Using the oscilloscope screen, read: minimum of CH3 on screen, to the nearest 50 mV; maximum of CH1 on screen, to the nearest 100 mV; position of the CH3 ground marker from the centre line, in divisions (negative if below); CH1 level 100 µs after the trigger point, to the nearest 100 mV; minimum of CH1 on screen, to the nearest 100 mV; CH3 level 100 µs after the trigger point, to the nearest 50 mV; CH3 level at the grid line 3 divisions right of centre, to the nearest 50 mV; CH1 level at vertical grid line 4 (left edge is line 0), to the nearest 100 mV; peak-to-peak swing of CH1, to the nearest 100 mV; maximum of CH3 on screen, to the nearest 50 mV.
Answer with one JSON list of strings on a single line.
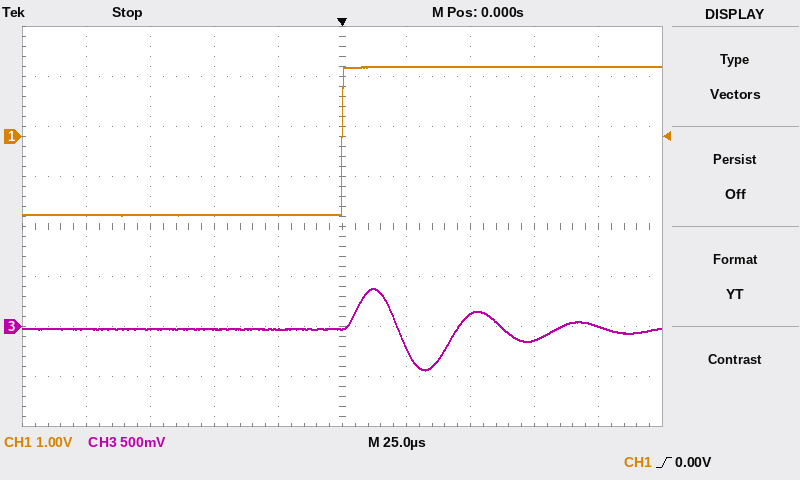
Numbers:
["-450 mV", "1.4 V", "-2.0 div", "1.4 V", "-1.6 V", "0 mV", "-150 mV", "-1.6 V", "3.0 V", "400 mV"]
